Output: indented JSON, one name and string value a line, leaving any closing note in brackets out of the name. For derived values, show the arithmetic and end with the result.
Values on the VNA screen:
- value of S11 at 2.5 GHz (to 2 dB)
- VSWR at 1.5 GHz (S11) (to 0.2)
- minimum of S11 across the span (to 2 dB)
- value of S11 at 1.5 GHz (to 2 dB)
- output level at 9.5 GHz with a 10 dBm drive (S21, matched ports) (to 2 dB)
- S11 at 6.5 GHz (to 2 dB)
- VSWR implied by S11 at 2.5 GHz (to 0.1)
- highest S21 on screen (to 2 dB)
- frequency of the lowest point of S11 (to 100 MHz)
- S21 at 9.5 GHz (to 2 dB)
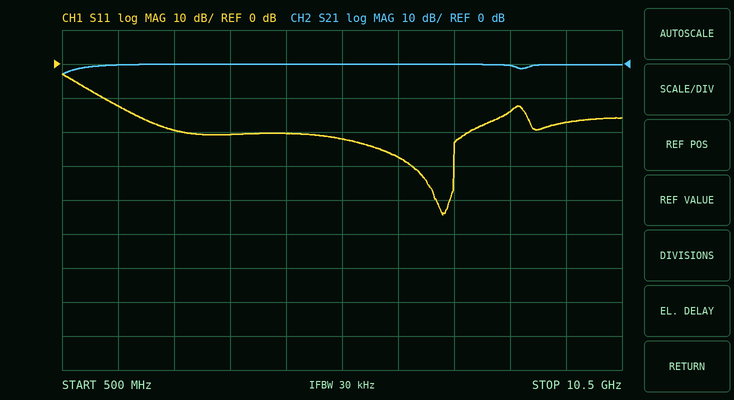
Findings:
{
  "value of S11 at 2.5 GHz": "-20 dB",
  "VSWR at 1.5 GHz (S11)": "|Γ| = 10^(-12/20) = 0.2512; VSWR = (1 + 0.2512)/(1 − 0.2512) ≈ 1.67, so 1.6 to the nearest 0.2",
  "minimum of S11 across the span": "-44 dB",
  "value of S11 at 1.5 GHz": "-12 dB",
  "output level at 9.5 GHz with a 10 dBm drive (S21, matched ports)": "10 dBm + (0 dB) = 10 dBm",
  "S11 at 6.5 GHz": "-28 dB",
  "VSWR implied by S11 at 2.5 GHz": "|Γ| = 10^(-20/20) = 0.1000; VSWR = (1 + 0.1000)/(1 − 0.1000) ≈ 1.2",
  "highest S21 on screen": "0 dB",
  "frequency of the lowest point of S11": "7.3 GHz",
  "S21 at 9.5 GHz": "0 dB"
}
